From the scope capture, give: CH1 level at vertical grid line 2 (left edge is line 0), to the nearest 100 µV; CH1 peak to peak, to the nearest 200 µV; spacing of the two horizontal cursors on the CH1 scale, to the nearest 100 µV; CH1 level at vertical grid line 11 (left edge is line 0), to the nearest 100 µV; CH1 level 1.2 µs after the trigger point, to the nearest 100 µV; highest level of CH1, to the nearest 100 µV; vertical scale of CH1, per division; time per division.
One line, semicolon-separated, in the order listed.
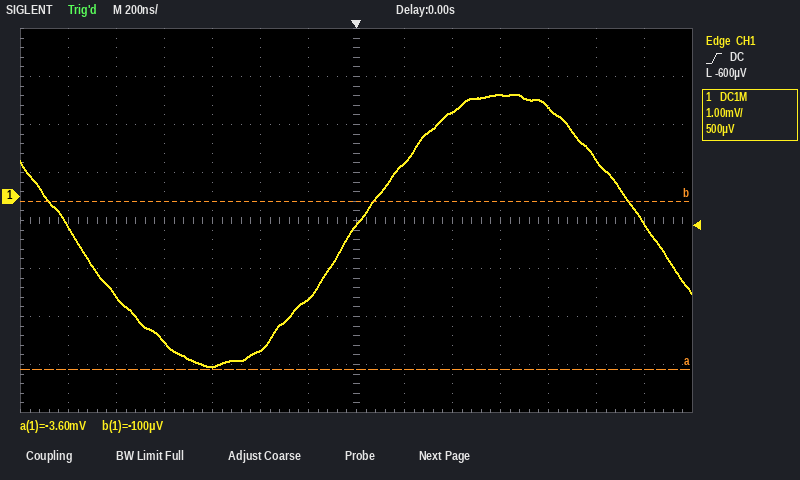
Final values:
-2.1 mV; 5.6 mV; 3.5 mV; 1.9 mV; -600 µV; 2.1 mV; 1 mV; 200 ns
